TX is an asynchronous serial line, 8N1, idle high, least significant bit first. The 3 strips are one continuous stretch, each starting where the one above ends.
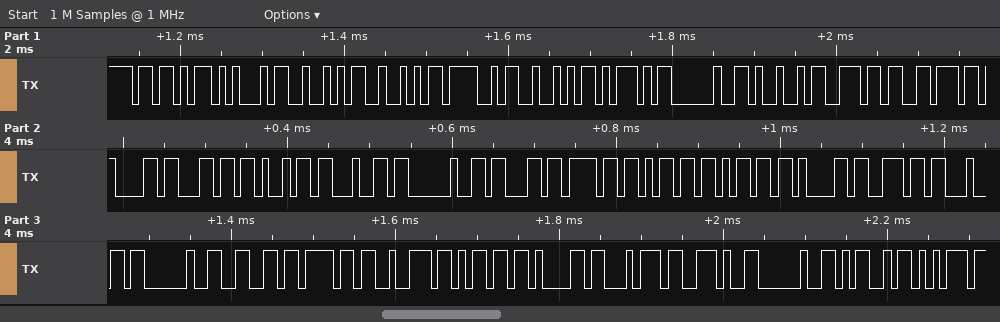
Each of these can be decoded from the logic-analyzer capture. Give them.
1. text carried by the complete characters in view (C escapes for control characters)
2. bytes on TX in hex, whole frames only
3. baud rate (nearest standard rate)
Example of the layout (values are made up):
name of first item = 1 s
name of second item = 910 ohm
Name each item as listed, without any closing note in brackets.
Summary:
text carried by the complete characters in view = "[ERROR] Invalid command format. Mu"
bytes on TX in hex, whole frames only = 5B 45 52 52 4F 52 5D 20 49 6E 76 61 6C 69 64 20 63 6F 6D 6D 61 6E 64 20 66 6F 72 6D 61 74 2E 20 4D 75
baud rate = 115200 baud
